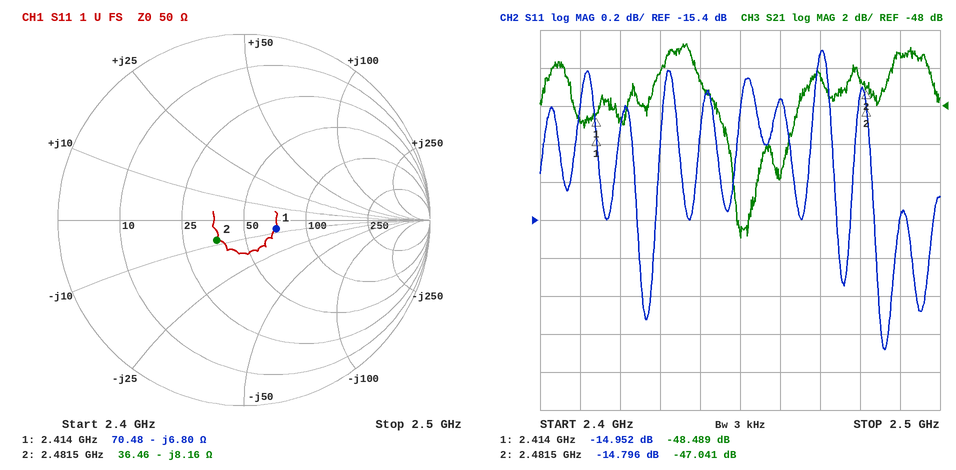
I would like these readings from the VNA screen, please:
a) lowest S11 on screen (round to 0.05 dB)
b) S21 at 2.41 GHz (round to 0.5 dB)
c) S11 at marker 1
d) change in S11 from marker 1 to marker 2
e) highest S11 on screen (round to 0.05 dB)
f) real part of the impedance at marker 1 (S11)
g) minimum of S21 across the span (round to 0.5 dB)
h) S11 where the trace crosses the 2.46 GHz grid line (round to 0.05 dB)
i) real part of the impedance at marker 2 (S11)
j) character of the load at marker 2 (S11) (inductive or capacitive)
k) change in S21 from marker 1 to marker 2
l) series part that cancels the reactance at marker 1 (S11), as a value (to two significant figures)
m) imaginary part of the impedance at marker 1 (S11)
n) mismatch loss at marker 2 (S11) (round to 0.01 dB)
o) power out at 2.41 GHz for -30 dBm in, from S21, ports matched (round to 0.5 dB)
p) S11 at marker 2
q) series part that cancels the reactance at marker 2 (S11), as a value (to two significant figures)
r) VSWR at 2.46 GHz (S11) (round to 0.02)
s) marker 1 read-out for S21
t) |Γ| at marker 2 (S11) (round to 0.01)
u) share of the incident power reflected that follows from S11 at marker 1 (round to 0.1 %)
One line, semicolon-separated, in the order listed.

-16.10 dB; -49.0 dB; -14.952 dB; 0.156 dB; -14.50 dB; 70.48 Ω; -55.0 dB; -14.75 dB; 36.46 Ω; capacitive; 1.448 dB; 450 pH; -6.80 Ω; 0.15 dB; -79.0 dBm; -14.796 dB; 520 pH; 1.44; -48.489 dB; 0.18; 3.2 %
